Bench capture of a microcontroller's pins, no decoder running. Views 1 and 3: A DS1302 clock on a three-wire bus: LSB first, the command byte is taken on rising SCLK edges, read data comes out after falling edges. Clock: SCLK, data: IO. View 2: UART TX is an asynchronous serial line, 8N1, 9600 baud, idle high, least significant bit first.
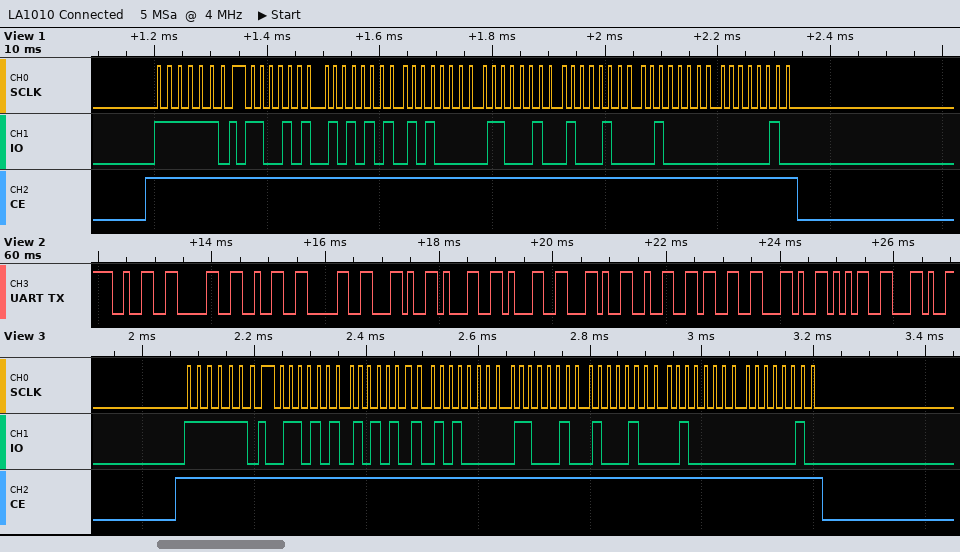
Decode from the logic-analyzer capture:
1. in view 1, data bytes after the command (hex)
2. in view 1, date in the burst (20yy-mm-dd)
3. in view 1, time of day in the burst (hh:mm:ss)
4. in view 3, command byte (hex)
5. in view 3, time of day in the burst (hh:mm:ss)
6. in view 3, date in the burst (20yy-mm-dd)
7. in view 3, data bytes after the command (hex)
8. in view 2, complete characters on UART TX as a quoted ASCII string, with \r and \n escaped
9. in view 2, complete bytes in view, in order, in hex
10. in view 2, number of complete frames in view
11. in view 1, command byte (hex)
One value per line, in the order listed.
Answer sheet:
53 55 05 23 11 02 20
2020-11-23
05:55:53
0xBF
05:55:56
2020-11-23
56 55 05 23 11 02 20
"2020,11,23,5,"
32 30 32 30 2C 31 31 2C 32 33 2C 35 2C
13
0xBF
